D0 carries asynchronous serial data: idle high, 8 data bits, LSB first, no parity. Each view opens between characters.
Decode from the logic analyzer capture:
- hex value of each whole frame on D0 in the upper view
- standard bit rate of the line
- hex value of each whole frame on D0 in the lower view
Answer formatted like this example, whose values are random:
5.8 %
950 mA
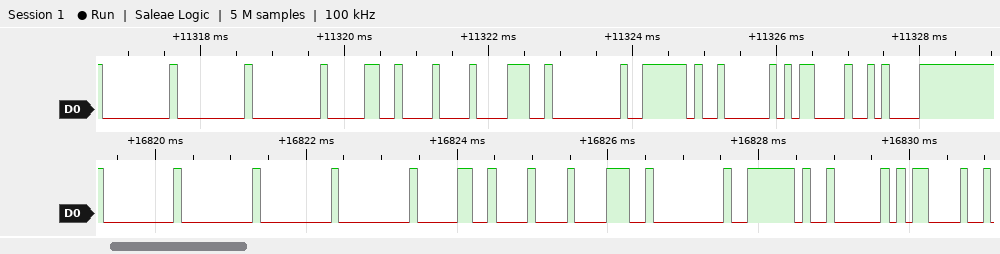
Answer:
00, 00, 00, 30, 08, 38, 00, 7E, 02, 0D, 0A
9600 baud
00, 00, 00, 00, 30, 08, 38, 00, 7E, 02, 0D
